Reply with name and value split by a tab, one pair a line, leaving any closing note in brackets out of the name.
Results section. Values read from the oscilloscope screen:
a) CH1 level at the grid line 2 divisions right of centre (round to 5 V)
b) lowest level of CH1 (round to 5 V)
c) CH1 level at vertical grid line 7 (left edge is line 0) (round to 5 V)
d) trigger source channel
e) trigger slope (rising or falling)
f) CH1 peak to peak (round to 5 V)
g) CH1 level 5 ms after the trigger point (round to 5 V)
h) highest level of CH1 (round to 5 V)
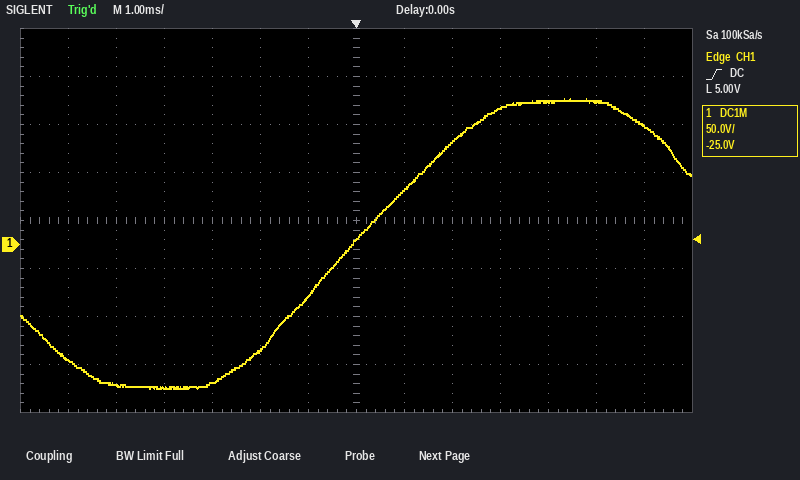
CH1 level at the grid line 2 divisions right of centre	105 V
lowest level of CH1	-150 V
CH1 level at vertical grid line 7 (left edge is line 0)	5 V
trigger source channel	CH1
trigger slope	rising
CH1 peak to peak	300 V
CH1 level 5 ms after the trigger point	150 V
highest level of CH1	150 V
